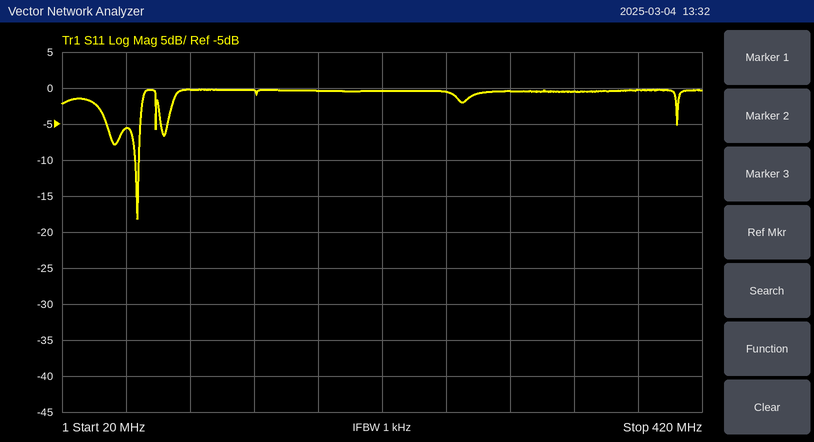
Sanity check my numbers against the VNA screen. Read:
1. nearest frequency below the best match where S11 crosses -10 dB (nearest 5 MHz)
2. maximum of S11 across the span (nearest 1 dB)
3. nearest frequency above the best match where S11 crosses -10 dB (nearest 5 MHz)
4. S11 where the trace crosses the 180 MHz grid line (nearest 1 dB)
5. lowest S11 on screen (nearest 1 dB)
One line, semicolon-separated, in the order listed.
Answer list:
65 MHz; 0 dB; 70 MHz; 0 dB; -18 dB
